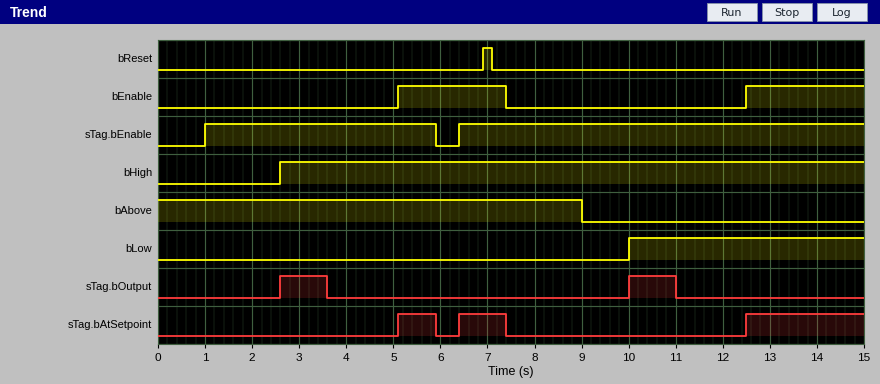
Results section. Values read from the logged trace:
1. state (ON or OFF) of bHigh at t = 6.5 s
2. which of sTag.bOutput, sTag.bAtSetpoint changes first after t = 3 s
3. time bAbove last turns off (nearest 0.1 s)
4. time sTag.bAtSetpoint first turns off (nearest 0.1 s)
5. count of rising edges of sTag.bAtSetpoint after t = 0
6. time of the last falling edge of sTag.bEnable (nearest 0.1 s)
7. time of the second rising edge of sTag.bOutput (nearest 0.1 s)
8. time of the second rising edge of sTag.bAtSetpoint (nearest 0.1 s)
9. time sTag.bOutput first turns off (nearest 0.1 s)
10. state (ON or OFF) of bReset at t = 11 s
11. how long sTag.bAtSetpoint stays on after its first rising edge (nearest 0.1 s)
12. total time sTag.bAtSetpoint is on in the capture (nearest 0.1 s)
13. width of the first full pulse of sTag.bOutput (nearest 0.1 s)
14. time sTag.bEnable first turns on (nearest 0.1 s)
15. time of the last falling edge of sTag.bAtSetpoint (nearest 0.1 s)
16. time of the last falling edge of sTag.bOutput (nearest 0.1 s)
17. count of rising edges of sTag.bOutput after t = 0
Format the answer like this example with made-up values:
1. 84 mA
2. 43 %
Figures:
1. ON
2. sTag.bOutput
3. 9.0 s
4. 5.9 s
5. 3
6. 5.9 s
7. 10.0 s
8. 6.4 s
9. 3.6 s
10. OFF
11. 0.8 s
12. 4.3 s
13. 1.0 s
14. 1.0 s
15. 7.4 s
16. 11.0 s
17. 2
